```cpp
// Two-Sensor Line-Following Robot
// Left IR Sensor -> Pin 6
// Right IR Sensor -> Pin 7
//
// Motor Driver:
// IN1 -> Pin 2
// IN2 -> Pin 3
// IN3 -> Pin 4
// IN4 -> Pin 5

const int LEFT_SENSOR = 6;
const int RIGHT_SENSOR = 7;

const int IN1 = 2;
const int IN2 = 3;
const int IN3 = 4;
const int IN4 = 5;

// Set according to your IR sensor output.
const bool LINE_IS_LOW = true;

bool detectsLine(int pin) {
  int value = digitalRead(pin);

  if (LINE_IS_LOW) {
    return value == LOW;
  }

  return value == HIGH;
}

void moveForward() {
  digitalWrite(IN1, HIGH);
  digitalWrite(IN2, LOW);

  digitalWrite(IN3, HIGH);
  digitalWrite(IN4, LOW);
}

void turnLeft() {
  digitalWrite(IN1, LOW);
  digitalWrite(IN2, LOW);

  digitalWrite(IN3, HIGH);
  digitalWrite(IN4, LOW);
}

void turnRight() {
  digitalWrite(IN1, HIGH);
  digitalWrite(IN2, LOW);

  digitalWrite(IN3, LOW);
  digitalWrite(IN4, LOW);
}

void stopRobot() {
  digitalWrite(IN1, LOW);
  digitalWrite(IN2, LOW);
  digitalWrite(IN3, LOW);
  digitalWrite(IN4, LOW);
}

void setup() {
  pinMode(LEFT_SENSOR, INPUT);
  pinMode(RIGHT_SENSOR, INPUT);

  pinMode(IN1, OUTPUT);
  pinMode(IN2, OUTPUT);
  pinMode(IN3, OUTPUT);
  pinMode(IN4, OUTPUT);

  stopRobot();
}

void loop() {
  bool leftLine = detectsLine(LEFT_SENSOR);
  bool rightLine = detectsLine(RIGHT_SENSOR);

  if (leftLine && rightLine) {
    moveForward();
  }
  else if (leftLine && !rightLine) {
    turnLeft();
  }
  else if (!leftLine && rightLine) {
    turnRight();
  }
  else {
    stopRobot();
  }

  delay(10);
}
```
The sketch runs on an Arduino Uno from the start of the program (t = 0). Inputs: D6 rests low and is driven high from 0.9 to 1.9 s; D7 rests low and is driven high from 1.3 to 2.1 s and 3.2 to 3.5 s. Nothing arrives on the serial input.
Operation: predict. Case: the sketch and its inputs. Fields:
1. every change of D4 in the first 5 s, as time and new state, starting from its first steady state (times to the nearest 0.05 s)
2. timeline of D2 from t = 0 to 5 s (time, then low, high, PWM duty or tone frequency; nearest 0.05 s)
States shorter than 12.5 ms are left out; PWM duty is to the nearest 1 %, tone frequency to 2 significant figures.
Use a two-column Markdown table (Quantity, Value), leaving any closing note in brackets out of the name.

| Quantity | Value |
|---|---|
| every change of D4 in the first 5 s, as time and new state, starting from its first steady state | 0 s high; 0.9 s low; 1.9 s high |
| timeline of D2 from t = 0 to 5 s | 0 s high; 1.3 s low; 2.1 s high; 3.2 s low; 3.5 s high |
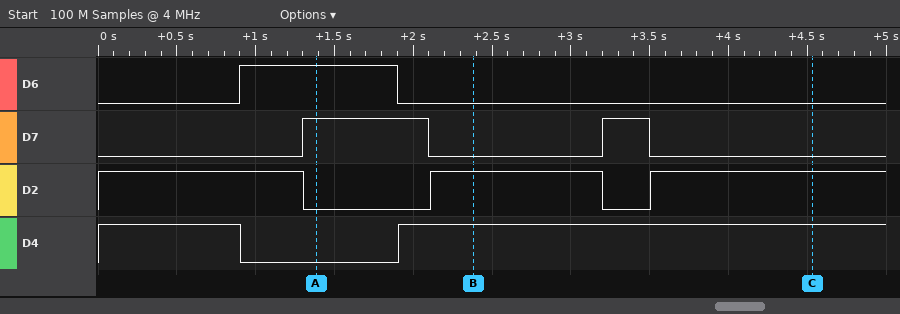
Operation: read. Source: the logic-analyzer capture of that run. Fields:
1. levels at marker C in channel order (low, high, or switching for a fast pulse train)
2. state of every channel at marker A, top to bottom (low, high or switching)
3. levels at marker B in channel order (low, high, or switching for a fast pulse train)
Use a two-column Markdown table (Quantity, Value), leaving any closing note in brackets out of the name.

| Quantity | Value |
|---|---|
| levels at marker C in channel order | D6 low, D7 low, D2 high, D4 high |
| state of every channel at marker A, top to bottom | D6 high, D7 high, D2 low, D4 low |
| levels at marker B in channel order | D6 low, D7 low, D2 high, D4 high |
